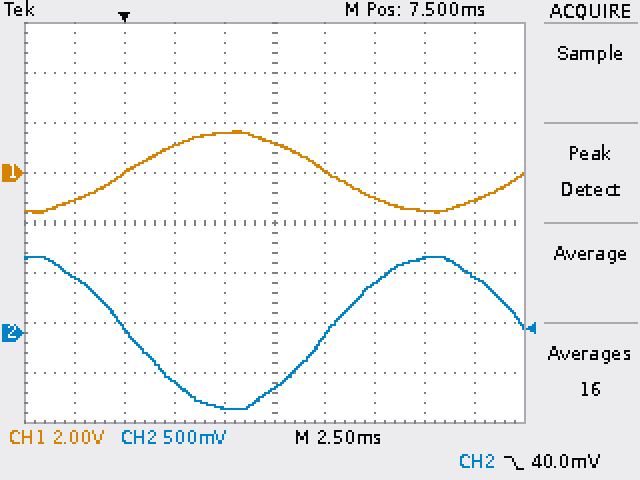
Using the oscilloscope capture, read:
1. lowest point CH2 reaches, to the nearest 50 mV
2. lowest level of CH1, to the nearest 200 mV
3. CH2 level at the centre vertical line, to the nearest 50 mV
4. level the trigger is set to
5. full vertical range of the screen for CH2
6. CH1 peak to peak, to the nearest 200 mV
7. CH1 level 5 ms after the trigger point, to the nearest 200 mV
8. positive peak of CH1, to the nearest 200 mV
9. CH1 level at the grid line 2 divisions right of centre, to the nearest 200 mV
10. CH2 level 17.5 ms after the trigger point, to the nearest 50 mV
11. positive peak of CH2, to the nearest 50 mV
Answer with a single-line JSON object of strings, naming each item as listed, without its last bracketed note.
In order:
{"lowest point CH2 reaches, to the nearest 50 mV": "-750 mV", "lowest level of CH1, to the nearest 200 mV": "-1.6 V", "CH2 level at the centre vertical line, to the nearest 50 mV": "-550 mV", "level the trigger is set to": "40.0 mV", "full vertical range of the screen for CH2": "4 V", "CH1 peak to peak, to the nearest 200 mV": "3.2 V", "CH1 level 5 ms after the trigger point, to the nearest 200 mV": "1.6 V", "positive peak of CH1, to the nearest 200 mV": "1.6 V", "CH1 level at the grid line 2 divisions right of centre, to the nearest 200 mV": "-1.0 V", "CH2 level 17.5 ms after the trigger point, to the nearest 50 mV": "550 mV", "positive peak of CH2, to the nearest 50 mV": "750 mV"}
